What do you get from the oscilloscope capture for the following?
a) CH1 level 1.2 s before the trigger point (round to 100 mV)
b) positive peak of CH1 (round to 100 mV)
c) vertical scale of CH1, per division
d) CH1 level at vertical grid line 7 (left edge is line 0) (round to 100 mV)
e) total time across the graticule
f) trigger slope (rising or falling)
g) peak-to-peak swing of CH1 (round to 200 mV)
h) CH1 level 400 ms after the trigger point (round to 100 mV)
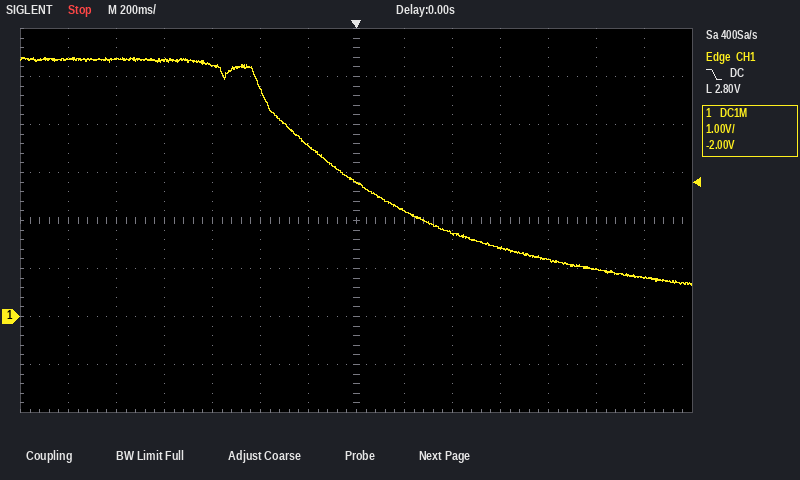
5.4 V
5.4 V
1 V
2.8 V
2.8 s
falling
4.8 V
1.7 V
